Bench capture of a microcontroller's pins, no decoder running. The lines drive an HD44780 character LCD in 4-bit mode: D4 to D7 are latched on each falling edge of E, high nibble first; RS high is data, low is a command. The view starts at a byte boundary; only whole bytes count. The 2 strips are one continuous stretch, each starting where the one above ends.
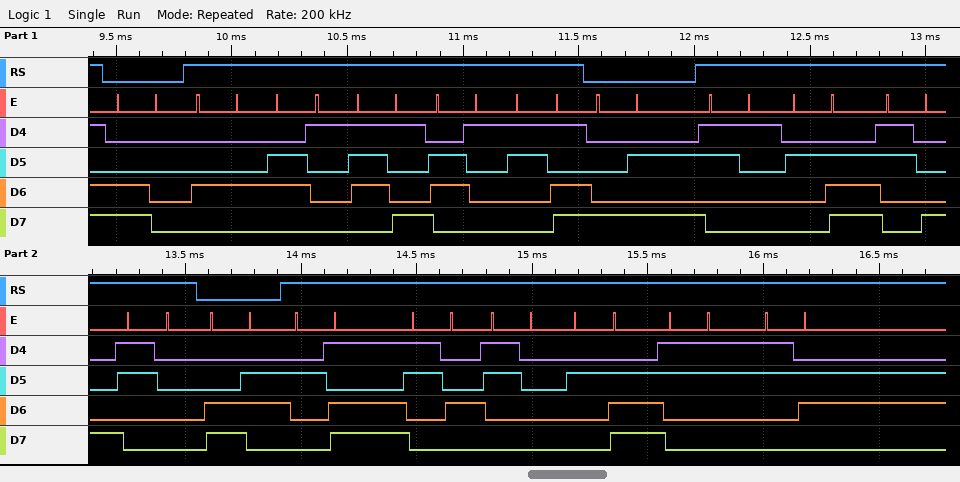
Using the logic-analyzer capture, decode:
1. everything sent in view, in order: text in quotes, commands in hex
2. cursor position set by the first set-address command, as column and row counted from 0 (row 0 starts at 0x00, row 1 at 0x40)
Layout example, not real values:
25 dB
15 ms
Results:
0xC0 "Daya=" 0x8A "1.80" 0xC6 "-40.36"
column 0, row 1
